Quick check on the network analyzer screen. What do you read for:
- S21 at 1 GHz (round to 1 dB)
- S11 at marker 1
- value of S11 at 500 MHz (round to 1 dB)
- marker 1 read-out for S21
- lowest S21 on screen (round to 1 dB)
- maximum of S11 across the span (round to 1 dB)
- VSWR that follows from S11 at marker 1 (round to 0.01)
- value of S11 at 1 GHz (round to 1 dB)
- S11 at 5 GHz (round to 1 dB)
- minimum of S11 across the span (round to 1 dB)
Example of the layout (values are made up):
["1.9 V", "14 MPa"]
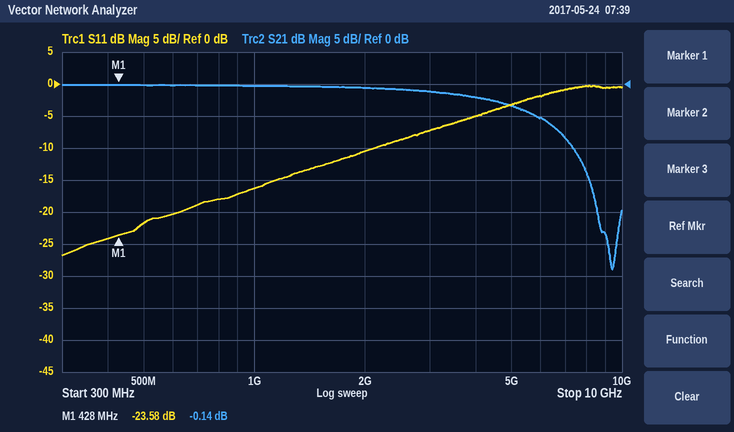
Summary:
["0 dB", "-23.58 dB", "-22 dB", "-0.14 dB", "-29 dB", "0 dB", "1.14", "-16 dB", "-3 dB", "-27 dB"]
